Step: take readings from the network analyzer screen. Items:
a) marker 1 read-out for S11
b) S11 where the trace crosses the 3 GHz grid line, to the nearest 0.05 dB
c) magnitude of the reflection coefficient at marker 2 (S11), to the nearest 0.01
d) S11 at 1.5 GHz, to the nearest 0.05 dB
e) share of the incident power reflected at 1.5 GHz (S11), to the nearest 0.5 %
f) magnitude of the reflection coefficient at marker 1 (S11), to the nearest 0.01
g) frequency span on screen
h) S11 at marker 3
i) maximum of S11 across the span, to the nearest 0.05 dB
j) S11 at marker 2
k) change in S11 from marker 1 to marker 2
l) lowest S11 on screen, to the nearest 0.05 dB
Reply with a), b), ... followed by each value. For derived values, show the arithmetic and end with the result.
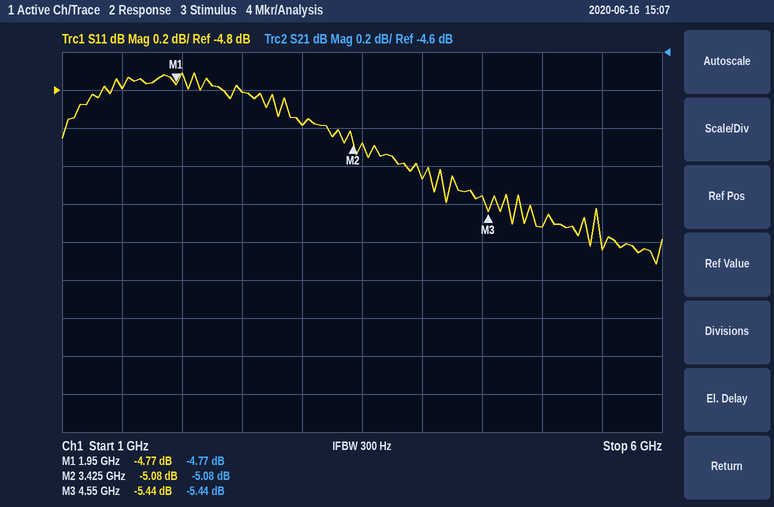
a) -4.77 dB
b) -5.00 dB
c) 10^(-5.08/20) ≈ 0.56
d) -4.80 dB
e) 10^(-4.8/10) ≈ 33.1 %, so 33.0 % to the nearest 0.5 %
f) 10^(-4.77/20) ≈ 0.58
g) 5 GHz
h) -5.44 dB
i) -4.70 dB
j) -5.08 dB
k) -5.08 − (-4.77) = -0.31 dB
l) -5.70 dB
